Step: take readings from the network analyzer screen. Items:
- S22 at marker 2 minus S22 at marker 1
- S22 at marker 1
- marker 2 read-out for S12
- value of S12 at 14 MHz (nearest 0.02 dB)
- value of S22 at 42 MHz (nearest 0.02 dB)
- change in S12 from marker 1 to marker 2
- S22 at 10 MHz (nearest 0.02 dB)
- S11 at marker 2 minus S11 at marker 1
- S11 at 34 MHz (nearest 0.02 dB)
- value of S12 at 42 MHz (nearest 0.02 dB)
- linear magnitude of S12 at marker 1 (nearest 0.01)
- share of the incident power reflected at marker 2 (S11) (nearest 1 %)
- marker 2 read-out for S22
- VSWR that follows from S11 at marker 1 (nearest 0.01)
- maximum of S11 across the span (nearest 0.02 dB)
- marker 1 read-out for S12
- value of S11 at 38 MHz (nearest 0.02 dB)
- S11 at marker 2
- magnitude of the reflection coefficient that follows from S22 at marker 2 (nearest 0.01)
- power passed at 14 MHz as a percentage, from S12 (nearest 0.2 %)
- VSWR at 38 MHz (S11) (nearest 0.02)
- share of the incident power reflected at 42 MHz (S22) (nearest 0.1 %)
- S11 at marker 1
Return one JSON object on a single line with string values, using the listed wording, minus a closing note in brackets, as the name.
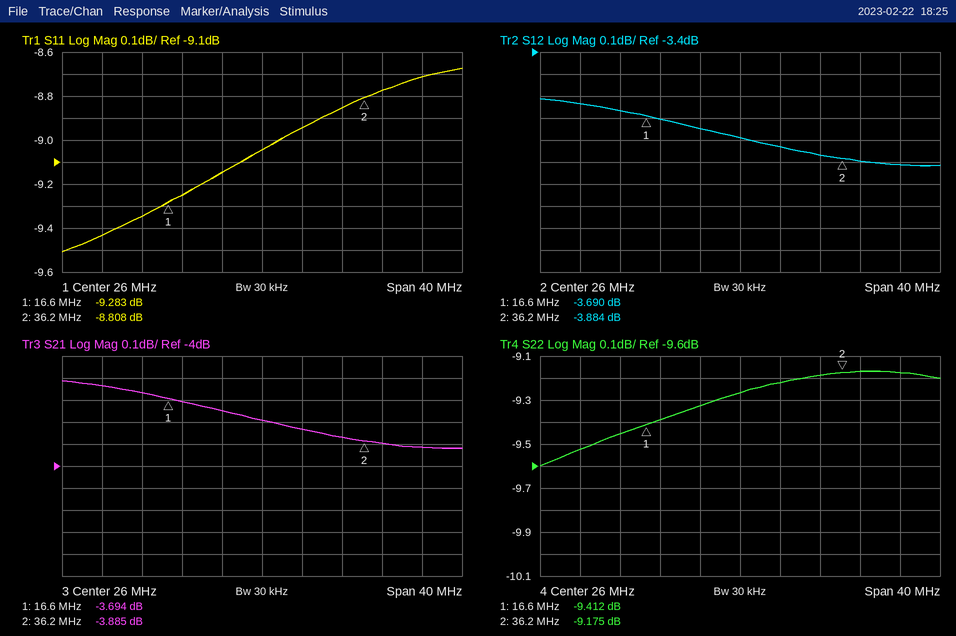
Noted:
{"S22 at marker 2 minus S22 at marker 1": "0.237 dB", "S22 at marker 1": "-9.412 dB", "marker 2 read-out for S12": "-3.884 dB", "value of S12 at 14 MHz": "-3.66 dB", "value of S22 at 42 MHz": "-9.18 dB", "change in S12 from marker 1 to marker 2": "-0.194 dB", "S22 at 10 MHz": "-9.52 dB", "S11 at marker 2 minus S11 at marker 1": "0.475 dB", "S11 at 34 MHz": "-8.86 dB", "value of S12 at 42 MHz": "-3.92 dB", "linear magnitude of S12 at marker 1": "0.65", "share of the incident power reflected at marker 2 (S11)": "13 %", "marker 2 read-out for S22": "-9.175 dB", "VSWR that follows from S11 at marker 1": "2.05", "maximum of S11 across the span": "-8.68 dB", "marker 1 read-out for S12": "-3.690 dB", "value of S11 at 38 MHz": "-8.78 dB", "S11 at marker 2": "-8.808 dB", "magnitude of the reflection coefficient that follows from S22 at marker 2": "0.35", "power passed at 14 MHz as a percentage, from S12": "43.0 %", "VSWR at 38 MHz (S11)": "2.14", "share of the incident power reflected at 42 MHz (S22)": "12.1 %", "S11 at marker 1": "-9.283 dB"}
